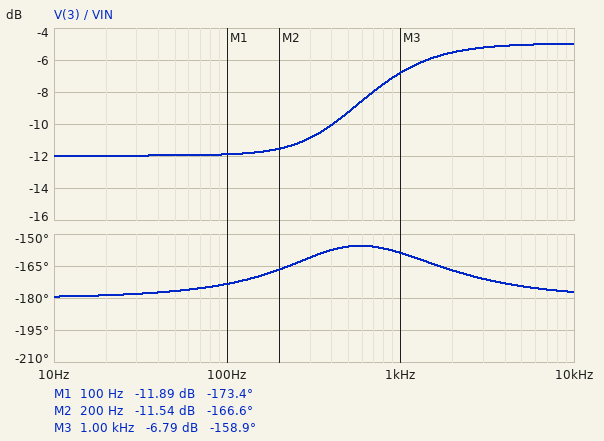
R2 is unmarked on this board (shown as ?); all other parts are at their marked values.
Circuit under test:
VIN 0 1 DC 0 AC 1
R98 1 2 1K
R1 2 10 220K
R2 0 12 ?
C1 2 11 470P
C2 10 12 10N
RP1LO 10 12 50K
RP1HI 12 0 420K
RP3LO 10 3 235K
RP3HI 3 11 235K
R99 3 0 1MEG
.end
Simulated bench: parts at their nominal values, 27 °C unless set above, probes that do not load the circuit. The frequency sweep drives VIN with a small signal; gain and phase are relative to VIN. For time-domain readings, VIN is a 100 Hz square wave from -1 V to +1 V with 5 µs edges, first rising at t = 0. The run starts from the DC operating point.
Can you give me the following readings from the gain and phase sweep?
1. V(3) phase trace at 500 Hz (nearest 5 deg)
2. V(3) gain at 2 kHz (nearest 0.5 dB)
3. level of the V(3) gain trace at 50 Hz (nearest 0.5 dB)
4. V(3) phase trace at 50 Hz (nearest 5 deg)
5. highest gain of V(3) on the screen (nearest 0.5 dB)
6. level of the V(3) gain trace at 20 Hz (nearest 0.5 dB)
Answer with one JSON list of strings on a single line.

["-155 deg", "-5.5 dB", "-12.0 dB", "-175 deg", "-5.0 dB", "-12.0 dB"]
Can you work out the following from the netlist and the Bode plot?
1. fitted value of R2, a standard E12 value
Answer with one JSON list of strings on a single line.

["68 kΩ"]
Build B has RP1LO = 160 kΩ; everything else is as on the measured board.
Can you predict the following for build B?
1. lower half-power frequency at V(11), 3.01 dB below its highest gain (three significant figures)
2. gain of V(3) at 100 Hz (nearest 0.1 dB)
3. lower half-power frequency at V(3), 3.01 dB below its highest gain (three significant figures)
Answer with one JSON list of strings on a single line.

["790 Hz", "-9.9 dB", "743 Hz"]
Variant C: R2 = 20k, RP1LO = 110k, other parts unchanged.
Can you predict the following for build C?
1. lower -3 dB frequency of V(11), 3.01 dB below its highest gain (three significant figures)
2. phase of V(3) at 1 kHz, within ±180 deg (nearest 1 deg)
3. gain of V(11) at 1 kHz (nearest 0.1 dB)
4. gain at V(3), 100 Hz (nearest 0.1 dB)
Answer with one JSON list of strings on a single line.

["863 Hz", "-154 deg", "-2.4 dB", "-12.0 dB"]
